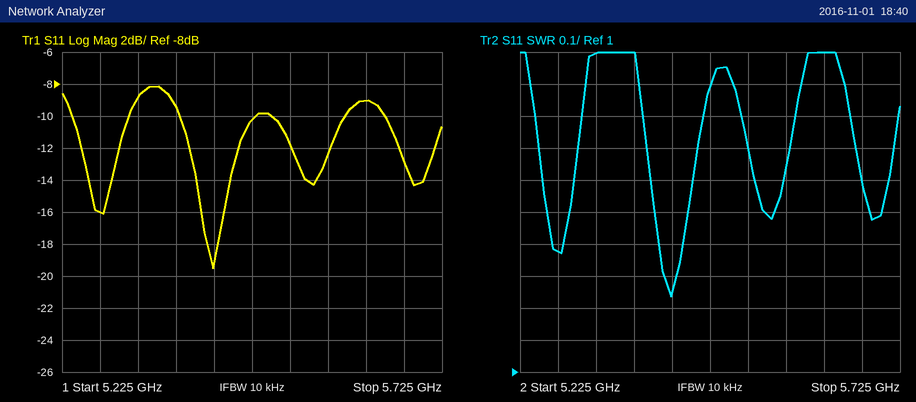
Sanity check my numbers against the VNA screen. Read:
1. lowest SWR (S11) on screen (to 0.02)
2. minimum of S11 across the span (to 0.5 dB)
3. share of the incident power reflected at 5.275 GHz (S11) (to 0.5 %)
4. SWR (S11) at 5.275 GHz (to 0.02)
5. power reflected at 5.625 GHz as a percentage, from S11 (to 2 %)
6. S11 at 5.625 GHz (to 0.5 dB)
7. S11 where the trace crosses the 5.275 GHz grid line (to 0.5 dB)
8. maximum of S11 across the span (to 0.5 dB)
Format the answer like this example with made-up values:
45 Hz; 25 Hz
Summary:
1.24; -19.5 dB; 2.5 %; 1.38; 12 %; -9.0 dB; -16.0 dB; -8.0 dB
